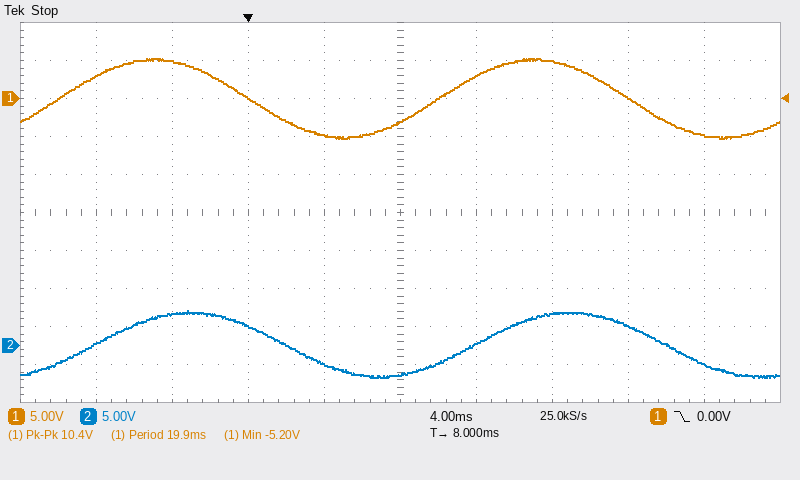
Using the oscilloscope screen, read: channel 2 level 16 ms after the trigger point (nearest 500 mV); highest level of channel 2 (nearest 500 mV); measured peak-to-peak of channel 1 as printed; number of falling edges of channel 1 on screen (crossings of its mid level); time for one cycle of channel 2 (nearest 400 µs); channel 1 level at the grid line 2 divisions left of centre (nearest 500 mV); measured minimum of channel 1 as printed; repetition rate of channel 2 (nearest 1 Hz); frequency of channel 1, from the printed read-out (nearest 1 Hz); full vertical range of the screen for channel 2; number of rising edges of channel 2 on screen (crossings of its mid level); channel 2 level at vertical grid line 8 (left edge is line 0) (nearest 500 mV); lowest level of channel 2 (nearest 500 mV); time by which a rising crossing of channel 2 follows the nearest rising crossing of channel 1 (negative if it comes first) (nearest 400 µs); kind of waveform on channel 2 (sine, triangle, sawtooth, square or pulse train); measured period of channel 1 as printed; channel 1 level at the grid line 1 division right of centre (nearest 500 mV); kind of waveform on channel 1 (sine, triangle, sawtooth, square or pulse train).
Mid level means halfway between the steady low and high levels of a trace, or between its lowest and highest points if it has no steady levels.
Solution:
4.0 V
4.5 V
10.4 V
2
20.0 ms
0.0 V
-5.20 V
50 Hz
50 Hz
50 V
2
2.5 V
-4.0 V
+2.0 ms
sine
19.9 ms
3.0 V
sine
